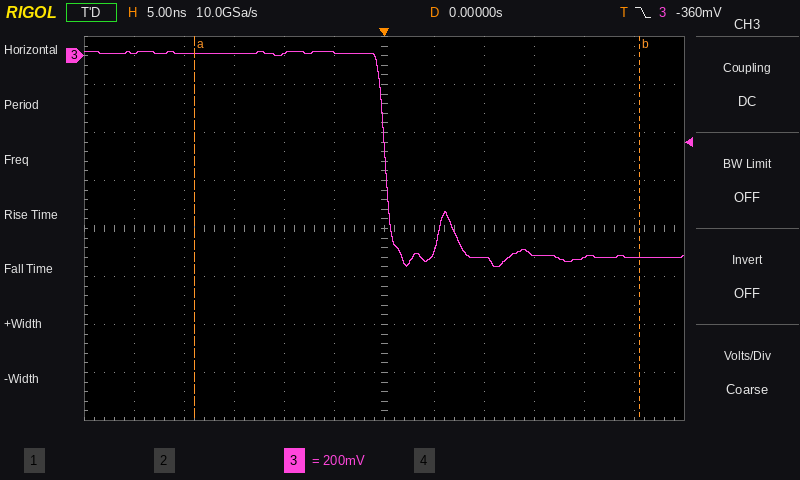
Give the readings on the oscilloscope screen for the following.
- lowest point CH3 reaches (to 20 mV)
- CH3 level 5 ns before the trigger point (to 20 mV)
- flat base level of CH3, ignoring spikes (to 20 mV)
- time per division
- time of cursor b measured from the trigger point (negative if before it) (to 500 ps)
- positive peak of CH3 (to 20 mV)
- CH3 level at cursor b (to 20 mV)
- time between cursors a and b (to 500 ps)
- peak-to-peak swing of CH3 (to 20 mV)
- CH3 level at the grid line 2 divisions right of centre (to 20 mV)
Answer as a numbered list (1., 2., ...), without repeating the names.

1. -880 mV
2. 20 mV
3. -840 mV
4. 5 ns
5. +25.5 ns
6. 20 mV
7. -840 mV
8. 44.5 ns
9. 900 mV
10. -840 mV
